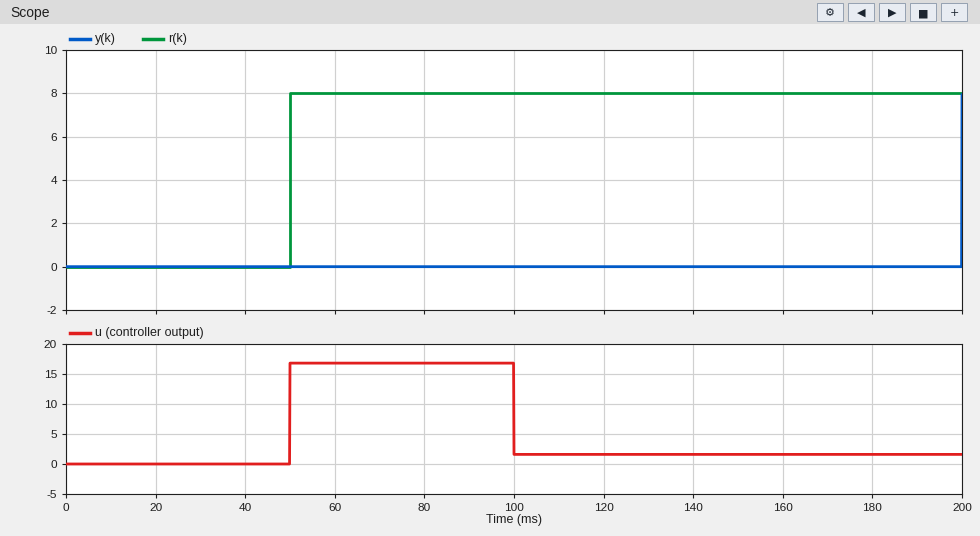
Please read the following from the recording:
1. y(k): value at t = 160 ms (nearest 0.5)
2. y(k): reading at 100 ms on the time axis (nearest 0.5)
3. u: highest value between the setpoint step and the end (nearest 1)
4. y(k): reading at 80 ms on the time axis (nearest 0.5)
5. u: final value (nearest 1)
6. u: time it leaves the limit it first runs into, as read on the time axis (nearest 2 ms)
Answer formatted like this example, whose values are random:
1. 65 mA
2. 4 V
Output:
1. 0.0
2. 0.0
3. 17
4. 0.0
5. 2
6. 100 ms
